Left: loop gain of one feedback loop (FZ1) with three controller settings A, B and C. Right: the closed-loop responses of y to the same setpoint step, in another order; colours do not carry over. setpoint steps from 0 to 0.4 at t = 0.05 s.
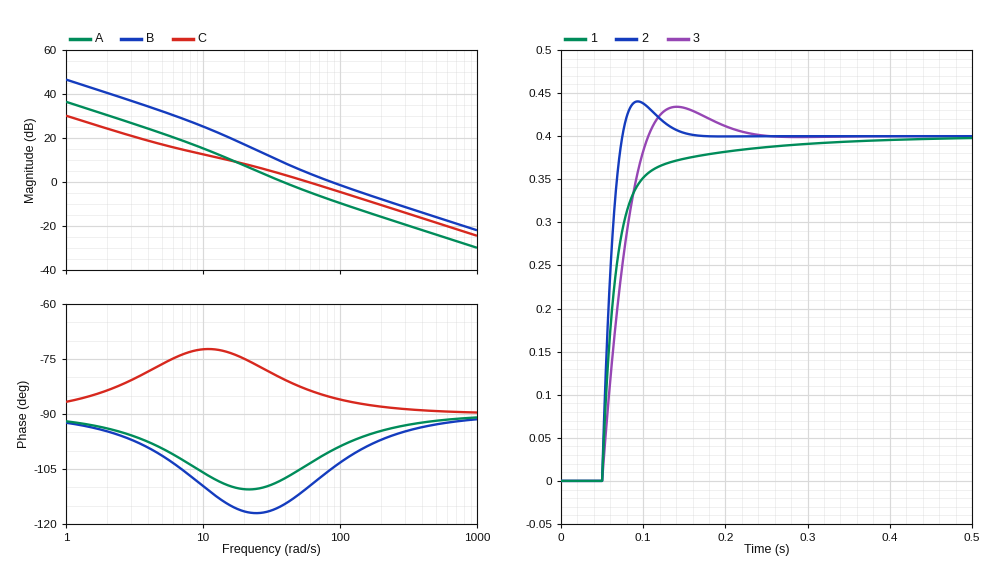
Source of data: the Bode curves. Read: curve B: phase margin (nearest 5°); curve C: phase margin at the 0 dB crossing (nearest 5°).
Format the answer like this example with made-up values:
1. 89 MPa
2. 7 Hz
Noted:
1. 75°
2. 95°
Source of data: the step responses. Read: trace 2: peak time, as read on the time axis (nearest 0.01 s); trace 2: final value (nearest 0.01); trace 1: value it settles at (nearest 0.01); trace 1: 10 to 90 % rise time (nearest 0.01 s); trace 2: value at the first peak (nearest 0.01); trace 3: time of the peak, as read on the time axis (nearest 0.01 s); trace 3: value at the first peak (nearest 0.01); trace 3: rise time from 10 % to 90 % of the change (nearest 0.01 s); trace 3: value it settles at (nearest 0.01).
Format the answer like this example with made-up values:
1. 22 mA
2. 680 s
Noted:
1. 0.09 s
2. 0.40
3. 0.40
4. 0.06 s
5. 0.44
6. 0.14 s
7. 0.43
8. 0.04 s
9. 0.40
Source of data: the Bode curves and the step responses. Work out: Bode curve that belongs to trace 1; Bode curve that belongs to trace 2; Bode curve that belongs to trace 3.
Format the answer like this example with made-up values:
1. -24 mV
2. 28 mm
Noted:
1. C
2. B
3. A
